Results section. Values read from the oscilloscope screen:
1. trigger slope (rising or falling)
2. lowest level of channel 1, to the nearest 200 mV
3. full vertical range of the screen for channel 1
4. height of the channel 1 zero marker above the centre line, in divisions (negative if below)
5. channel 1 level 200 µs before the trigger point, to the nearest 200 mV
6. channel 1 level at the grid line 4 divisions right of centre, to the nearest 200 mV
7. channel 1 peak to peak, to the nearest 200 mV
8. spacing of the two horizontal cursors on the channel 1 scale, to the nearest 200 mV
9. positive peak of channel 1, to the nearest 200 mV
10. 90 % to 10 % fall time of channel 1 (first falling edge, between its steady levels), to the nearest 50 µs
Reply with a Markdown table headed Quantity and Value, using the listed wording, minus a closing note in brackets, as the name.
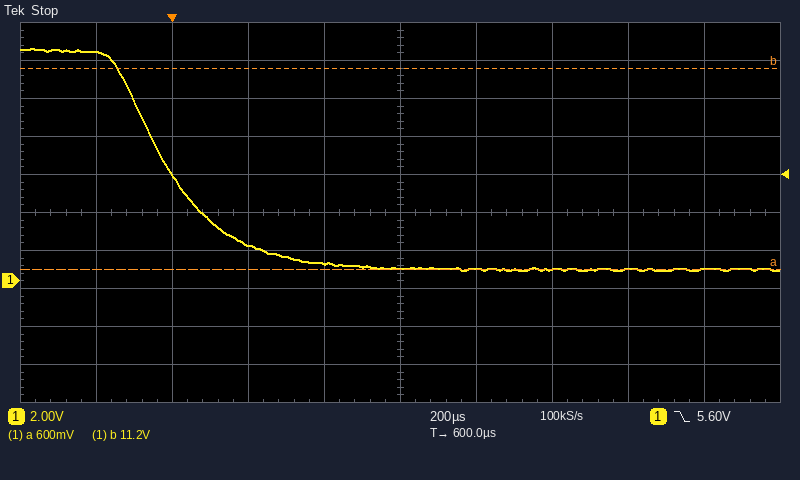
| Quantity | Value |
|---|---|
| trigger slope | falling |
| lowest level of channel 1, to the nearest 200 mV | 600 mV |
| full vertical range of the screen for channel 1 | 20 V |
| height of the channel 1 zero marker above the centre line, in divisions | -1.8 div |
| channel 1 level 200 µs before the trigger point, to the nearest 200 mV | 12.0 V |
| channel 1 level at the grid line 4 divisions right of centre, to the nearest 200 mV | 600 mV |
| channel 1 peak to peak, to the nearest 200 mV | 11.6 V |
| spacing of the two horizontal cursors on the channel 1 scale, to the nearest 200 mV | 10.6 V |
| positive peak of channel 1, to the nearest 200 mV | 12.2 V |
| 90 % to 10 % fall time of channel 1 (first falling edge, between its steady levels), to the nearest 50 µs | 350 µs |
